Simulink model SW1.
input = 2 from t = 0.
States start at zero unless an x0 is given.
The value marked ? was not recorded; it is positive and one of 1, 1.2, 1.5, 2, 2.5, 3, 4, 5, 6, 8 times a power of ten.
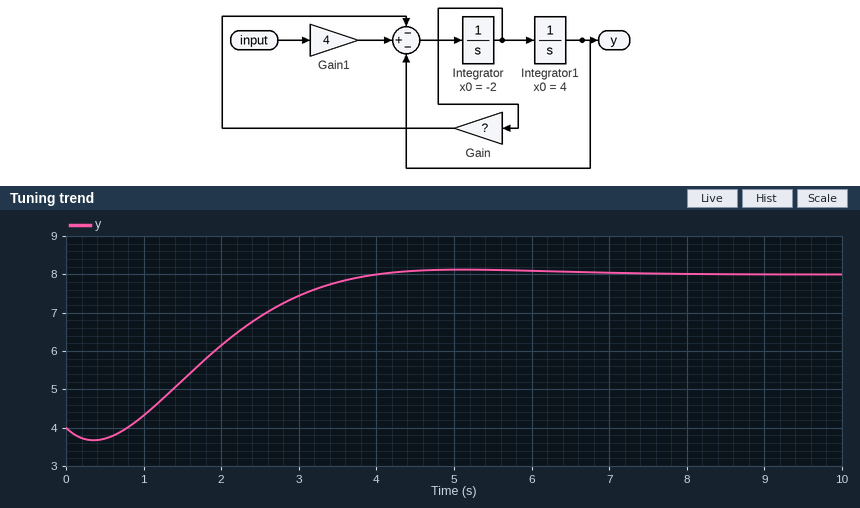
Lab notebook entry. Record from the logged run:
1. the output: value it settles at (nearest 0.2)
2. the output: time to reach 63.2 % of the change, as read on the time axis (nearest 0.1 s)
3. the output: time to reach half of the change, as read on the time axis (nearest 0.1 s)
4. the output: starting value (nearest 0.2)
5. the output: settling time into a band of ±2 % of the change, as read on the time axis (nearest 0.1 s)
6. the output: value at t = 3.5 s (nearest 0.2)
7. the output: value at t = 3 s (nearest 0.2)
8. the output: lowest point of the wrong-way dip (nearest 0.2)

8.0
2.2 s
1.9 s
4.0
6.2 s
7.8
7.4
3.6
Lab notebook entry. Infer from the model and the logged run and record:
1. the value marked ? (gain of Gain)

1.5
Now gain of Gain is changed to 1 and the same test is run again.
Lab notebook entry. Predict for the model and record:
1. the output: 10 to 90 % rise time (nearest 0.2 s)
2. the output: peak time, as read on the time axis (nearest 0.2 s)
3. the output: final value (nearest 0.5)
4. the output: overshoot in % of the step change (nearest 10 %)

1.4 s
4.0 s
8.0
20 %
